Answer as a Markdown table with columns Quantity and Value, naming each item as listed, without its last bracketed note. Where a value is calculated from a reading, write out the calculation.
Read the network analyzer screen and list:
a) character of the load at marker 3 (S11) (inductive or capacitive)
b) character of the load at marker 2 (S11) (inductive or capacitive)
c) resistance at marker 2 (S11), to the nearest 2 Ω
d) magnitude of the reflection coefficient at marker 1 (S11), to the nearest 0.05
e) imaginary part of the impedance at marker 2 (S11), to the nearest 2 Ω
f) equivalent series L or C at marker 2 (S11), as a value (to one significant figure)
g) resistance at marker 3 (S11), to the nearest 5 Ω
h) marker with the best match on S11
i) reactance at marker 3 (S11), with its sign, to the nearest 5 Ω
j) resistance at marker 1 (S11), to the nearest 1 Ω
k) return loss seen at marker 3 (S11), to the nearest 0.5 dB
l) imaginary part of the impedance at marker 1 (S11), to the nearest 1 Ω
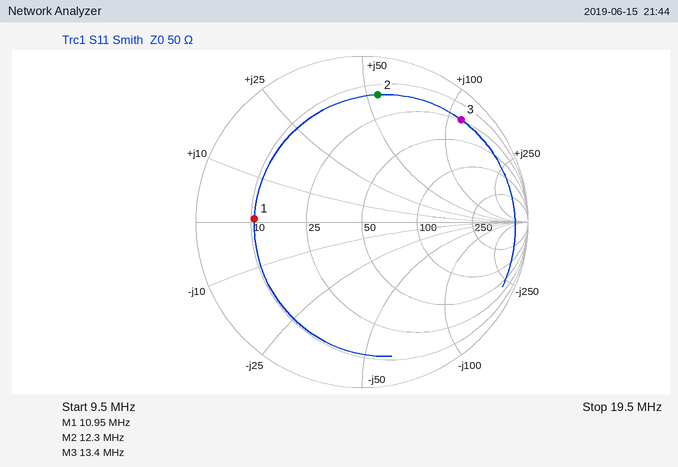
| Quantity | Value |
|---|---|
| character of the load at marker 3 (S11) | inductive |
| character of the load at marker 2 (S11) | inductive |
| resistance at marker 2 (S11), to the nearest 2 Ω | 14 Ω |
| magnitude of the reflection coefficient at marker 1 (S11), to the nearest 0.05 | 0.65 |
| imaginary part of the impedance at marker 2 (S11), to the nearest 2 Ω | +54 Ω |
| equivalent series L or C at marker 2 (S11), as a value | L = 54 Ω/(2π × 12.3 MHz) ≈ 699 nH, so 700 nH to one significant figure |
| resistance at marker 3 (S11), to the nearest 5 Ω | 25 Ω |
| marker with the best match on S11 | marker 1 |
| reactance at marker 3 (S11), with its sign, to the nearest 5 Ω | +115 Ω |
| resistance at marker 1 (S11), to the nearest 1 Ω | 11 Ω |
| return loss seen at marker 3 (S11), to the nearest 0.5 dB | 1.5 dB |
| imaginary part of the impedance at marker 1 (S11), to the nearest 1 Ω | +1 Ω |
